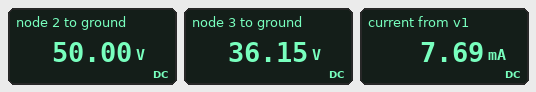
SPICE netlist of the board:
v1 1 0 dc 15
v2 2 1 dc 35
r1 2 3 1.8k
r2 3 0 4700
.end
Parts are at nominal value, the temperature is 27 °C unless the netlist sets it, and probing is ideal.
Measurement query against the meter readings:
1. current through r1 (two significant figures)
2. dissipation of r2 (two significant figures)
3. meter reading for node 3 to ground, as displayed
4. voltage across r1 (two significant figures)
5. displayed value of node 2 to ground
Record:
7.7 mA
280 mW
36.15 V
14 V
50.00 V
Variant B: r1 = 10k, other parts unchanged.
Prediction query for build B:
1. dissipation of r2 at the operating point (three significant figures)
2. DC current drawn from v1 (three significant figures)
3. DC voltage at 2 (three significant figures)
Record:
54.4 mW
3.40 mA
50.0 V
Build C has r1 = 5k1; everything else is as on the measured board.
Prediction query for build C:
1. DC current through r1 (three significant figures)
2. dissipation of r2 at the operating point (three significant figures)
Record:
5.10 mA
122 mW
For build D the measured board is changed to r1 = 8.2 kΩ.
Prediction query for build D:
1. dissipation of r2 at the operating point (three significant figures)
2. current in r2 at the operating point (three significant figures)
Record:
70.6 mW
3.88 mA
